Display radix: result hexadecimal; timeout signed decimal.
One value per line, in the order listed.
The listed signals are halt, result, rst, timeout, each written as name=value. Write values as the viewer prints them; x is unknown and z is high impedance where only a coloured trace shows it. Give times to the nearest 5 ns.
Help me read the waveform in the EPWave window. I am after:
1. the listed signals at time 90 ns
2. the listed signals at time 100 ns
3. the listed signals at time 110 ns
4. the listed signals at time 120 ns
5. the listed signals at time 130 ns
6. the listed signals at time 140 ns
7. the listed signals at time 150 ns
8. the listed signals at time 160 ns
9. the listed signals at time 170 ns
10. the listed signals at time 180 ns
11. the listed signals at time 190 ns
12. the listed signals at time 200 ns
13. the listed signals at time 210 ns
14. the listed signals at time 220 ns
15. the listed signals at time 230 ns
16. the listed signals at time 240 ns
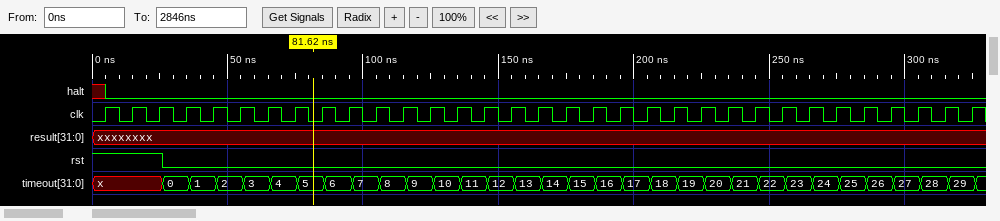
halt=0, result=xxxxxxxx, rst=0, timeout=6
halt=0, result=xxxxxxxx, rst=0, timeout=7
halt=0, result=xxxxxxxx, rst=0, timeout=8
halt=0, result=xxxxxxxx, rst=0, timeout=9
halt=0, result=xxxxxxxx, rst=0, timeout=10
halt=0, result=xxxxxxxx, rst=0, timeout=11
halt=0, result=xxxxxxxx, rst=0, timeout=12
halt=0, result=xxxxxxxx, rst=0, timeout=13
halt=0, result=xxxxxxxx, rst=0, timeout=14
halt=0, result=xxxxxxxx, rst=0, timeout=15
halt=0, result=xxxxxxxx, rst=0, timeout=16
halt=0, result=xxxxxxxx, rst=0, timeout=17
halt=0, result=xxxxxxxx, rst=0, timeout=18
halt=0, result=xxxxxxxx, rst=0, timeout=19
halt=0, result=xxxxxxxx, rst=0, timeout=20
halt=0, result=xxxxxxxx, rst=0, timeout=21
